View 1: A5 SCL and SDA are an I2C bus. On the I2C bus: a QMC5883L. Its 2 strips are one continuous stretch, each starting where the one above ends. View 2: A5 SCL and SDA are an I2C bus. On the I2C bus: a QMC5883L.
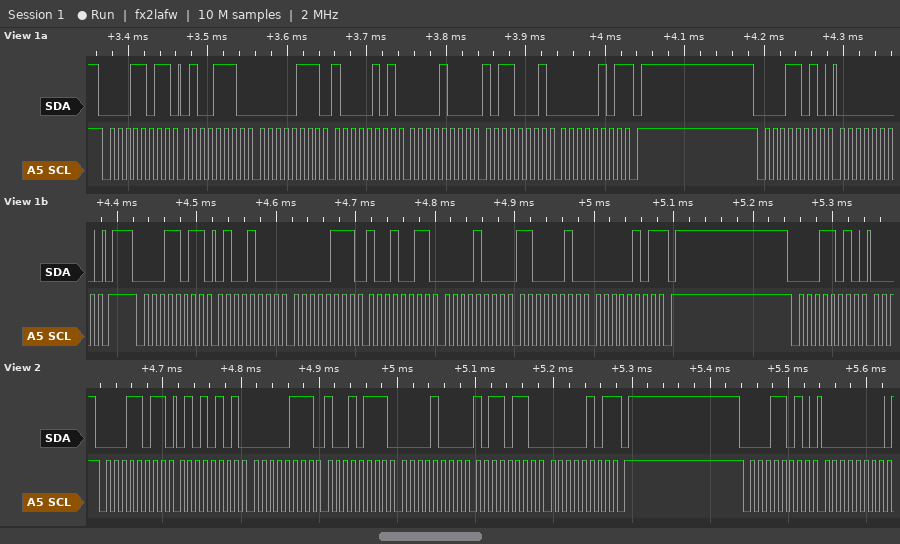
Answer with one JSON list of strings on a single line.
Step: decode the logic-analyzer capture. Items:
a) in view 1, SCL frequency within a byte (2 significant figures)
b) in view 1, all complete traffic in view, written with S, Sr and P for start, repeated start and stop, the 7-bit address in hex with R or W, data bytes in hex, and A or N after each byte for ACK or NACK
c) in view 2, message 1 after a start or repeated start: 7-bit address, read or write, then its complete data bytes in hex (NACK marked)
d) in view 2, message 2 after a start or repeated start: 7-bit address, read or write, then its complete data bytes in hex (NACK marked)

["100 kHz", "S 0DR A 4E A 07 A 85 A 08 A B1 A 05 N P S 0DW A 00 A P S 0DR A 48 A 07 A 93 A 08 A C2 A 05 N P S 0DW A", "0x0D read: 55 07 97 08 B6 05 NACK", "0x0D write: 00"]
